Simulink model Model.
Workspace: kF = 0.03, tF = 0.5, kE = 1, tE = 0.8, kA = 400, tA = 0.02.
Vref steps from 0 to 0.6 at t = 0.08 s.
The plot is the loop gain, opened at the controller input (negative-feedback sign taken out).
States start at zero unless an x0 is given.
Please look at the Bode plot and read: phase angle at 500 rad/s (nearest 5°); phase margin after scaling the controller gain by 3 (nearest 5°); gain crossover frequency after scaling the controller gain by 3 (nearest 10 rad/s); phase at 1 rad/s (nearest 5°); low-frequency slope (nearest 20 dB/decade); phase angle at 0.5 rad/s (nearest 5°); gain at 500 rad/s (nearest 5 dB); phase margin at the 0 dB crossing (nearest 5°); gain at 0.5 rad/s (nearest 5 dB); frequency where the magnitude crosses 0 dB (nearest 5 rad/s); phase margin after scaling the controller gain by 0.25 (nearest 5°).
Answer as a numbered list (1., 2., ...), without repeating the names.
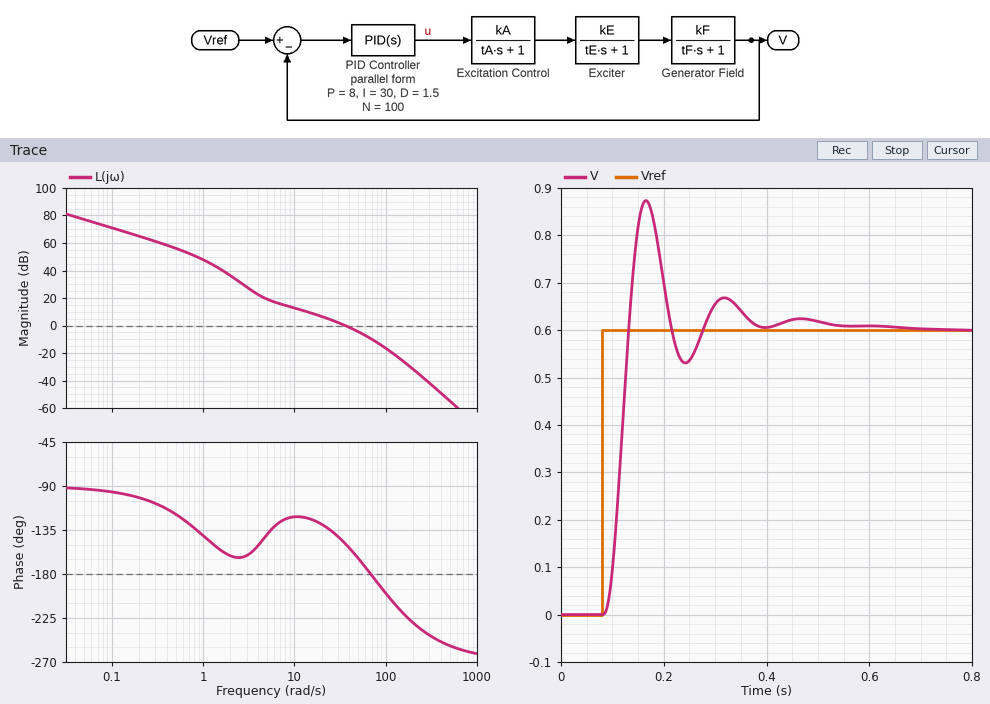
1. -255°
2. 0°
3. 70 rad/s
4. -140°
5. -20 dB/decade
6. -120°
7. -55 dB
8. 30°
9. 55 dB
10. 35 rad/s
11. 60°
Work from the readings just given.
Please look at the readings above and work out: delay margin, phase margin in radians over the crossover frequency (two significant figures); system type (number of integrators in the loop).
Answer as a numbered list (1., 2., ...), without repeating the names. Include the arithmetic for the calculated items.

1. 30 × π / 180 / 35 = 0.015 s
2. 1
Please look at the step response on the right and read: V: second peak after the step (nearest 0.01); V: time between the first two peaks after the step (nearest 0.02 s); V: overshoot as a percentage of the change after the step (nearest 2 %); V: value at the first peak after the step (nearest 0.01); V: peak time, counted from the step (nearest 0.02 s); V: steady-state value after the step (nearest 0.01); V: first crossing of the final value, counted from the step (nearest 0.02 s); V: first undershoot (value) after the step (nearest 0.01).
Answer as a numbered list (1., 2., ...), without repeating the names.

1. 0.67
2. 0.16 s
3. 46 %
4. 0.87
5. 0.08 s
6. 0.60
7. 0.06 s
8. 0.53
